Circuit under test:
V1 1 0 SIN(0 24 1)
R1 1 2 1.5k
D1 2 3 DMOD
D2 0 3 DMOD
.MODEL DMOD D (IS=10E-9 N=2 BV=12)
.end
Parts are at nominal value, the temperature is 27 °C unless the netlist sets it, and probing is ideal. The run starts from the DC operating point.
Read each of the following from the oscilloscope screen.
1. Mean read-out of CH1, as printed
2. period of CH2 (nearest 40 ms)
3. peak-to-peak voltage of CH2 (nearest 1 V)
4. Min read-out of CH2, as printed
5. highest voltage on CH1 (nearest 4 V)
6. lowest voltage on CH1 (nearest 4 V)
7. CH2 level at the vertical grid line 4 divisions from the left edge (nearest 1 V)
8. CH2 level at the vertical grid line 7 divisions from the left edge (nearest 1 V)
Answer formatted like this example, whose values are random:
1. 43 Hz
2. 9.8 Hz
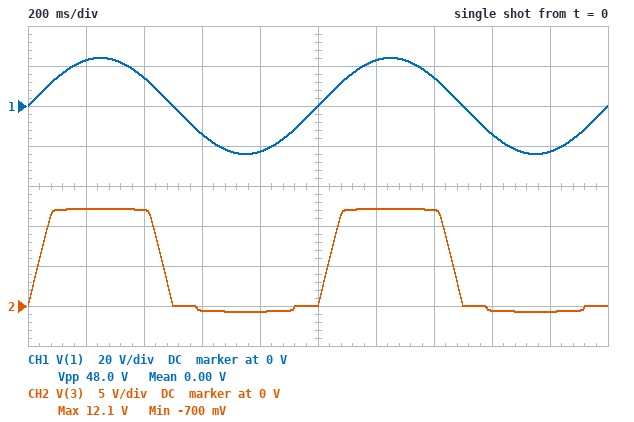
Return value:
1. 0.00 V
2. 1.00 s
3. 13 V
4. -700 mV
5. 24 V
6. -24 V
7. -1 V
8. 12 V
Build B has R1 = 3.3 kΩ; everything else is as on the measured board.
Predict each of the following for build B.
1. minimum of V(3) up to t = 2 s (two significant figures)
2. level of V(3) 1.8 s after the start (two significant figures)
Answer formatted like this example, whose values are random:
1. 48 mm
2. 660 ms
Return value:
1. -660 mV
2. -650 mV
